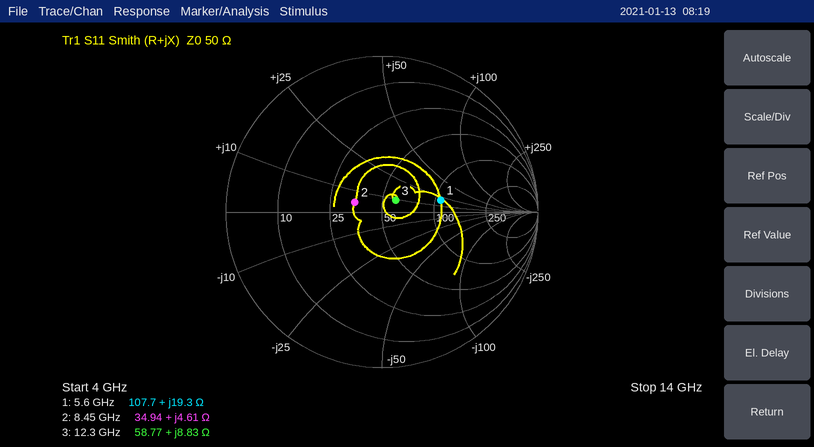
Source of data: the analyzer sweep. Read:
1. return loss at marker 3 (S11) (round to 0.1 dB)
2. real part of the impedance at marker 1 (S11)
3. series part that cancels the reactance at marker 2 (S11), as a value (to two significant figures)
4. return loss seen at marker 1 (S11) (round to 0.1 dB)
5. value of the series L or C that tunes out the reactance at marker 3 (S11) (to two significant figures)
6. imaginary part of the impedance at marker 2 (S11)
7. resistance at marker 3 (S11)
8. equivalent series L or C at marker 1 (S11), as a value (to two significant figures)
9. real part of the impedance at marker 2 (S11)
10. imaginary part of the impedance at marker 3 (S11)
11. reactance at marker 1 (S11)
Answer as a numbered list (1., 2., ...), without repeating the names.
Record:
1. 18.9 dB
2. 107.7 Ω
3. 4.1 pF
4. 8.3 dB
5. 1.5 pF
6. +4.61 Ω
7. 58.77 Ω
8. 550 pH
9. 34.94 Ω
10. +8.83 Ω
11. +19.3 Ω
